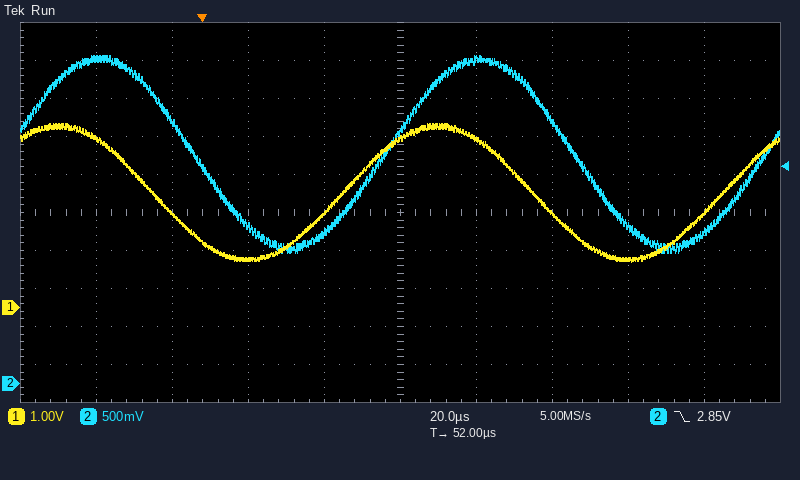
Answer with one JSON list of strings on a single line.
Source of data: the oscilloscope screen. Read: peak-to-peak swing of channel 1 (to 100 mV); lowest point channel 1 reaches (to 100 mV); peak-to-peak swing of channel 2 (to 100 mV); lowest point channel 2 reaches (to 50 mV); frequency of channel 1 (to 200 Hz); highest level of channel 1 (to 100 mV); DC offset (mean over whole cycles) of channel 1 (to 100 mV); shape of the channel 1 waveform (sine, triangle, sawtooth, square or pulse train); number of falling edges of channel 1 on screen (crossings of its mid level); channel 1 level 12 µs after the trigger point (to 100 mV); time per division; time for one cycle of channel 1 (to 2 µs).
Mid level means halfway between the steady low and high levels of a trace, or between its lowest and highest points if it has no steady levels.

["3.6 V", "1.2 V", "2.60 V", "1.70 V", "10.0 kHz", "4.8 V", "3.0 V", "sine", "2", "1.3 V", "20 µs", "100 µs"]
